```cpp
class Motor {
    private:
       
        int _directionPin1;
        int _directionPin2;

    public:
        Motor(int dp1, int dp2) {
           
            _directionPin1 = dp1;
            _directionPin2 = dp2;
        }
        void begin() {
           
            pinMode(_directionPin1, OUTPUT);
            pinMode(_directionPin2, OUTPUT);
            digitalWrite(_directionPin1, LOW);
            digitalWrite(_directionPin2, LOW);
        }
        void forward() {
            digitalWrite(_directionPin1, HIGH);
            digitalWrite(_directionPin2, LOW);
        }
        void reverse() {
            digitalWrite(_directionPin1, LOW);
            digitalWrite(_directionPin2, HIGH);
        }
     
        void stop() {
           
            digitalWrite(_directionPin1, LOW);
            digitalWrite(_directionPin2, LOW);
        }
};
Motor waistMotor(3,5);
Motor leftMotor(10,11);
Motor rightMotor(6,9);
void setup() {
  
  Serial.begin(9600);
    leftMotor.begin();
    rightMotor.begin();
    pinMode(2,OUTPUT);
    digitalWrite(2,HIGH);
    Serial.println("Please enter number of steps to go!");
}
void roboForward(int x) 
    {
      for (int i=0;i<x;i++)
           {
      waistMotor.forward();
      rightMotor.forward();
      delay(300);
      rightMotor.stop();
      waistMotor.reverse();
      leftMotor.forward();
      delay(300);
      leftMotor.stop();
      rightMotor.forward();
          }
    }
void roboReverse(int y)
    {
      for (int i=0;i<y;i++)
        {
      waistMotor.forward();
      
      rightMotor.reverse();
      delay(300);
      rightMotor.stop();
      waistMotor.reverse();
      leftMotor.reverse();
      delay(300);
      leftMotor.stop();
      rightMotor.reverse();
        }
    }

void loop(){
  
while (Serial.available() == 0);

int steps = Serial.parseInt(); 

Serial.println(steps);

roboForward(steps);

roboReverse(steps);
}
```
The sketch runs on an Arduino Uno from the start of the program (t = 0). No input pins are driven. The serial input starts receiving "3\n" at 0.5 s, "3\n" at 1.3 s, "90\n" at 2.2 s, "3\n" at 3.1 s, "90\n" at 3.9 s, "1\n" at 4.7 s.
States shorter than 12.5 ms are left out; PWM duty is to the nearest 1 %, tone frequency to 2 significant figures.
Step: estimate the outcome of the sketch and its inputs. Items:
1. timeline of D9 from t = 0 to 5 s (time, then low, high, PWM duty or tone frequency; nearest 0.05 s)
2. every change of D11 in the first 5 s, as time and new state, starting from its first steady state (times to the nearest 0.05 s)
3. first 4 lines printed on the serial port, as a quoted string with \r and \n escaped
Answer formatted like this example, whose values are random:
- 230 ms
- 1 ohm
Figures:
- 0 s low; 2.3 s high; 2.6 s low; 2.9 s high; 3.2 s low; 3.5 s high; 3.8 s low
- 0 s low; 2.6 s high; 2.9 s low; 3.2 s high; 3.5 s low; 3.8 s high; 4.1 s low
- "Please enter number of steps to go!\r\n3\r\n3\r\n90\r\n"
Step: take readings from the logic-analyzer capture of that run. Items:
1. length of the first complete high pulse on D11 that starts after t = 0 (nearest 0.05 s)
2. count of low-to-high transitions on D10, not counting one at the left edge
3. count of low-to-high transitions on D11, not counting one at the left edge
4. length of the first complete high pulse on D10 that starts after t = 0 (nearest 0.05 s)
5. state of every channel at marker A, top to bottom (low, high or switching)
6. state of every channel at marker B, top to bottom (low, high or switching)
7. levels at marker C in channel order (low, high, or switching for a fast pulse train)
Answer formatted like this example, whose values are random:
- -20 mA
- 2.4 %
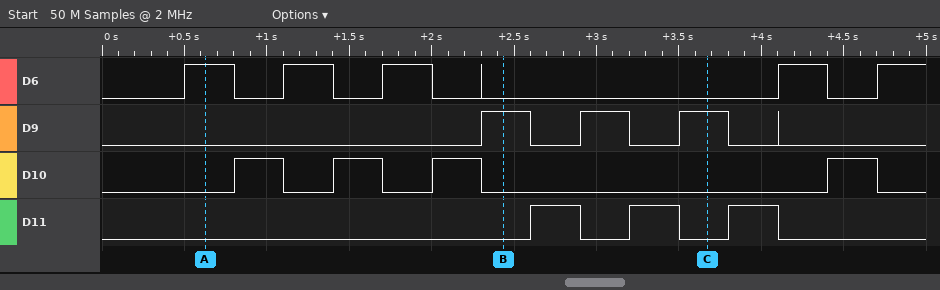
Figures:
- 0.30 s
- 4
- 3
- 0.30 s
- D6 high, D9 low, D10 low, D11 low
- D6 low, D9 high, D10 low, D11 low
- D6 low, D9 high, D10 low, D11 low
